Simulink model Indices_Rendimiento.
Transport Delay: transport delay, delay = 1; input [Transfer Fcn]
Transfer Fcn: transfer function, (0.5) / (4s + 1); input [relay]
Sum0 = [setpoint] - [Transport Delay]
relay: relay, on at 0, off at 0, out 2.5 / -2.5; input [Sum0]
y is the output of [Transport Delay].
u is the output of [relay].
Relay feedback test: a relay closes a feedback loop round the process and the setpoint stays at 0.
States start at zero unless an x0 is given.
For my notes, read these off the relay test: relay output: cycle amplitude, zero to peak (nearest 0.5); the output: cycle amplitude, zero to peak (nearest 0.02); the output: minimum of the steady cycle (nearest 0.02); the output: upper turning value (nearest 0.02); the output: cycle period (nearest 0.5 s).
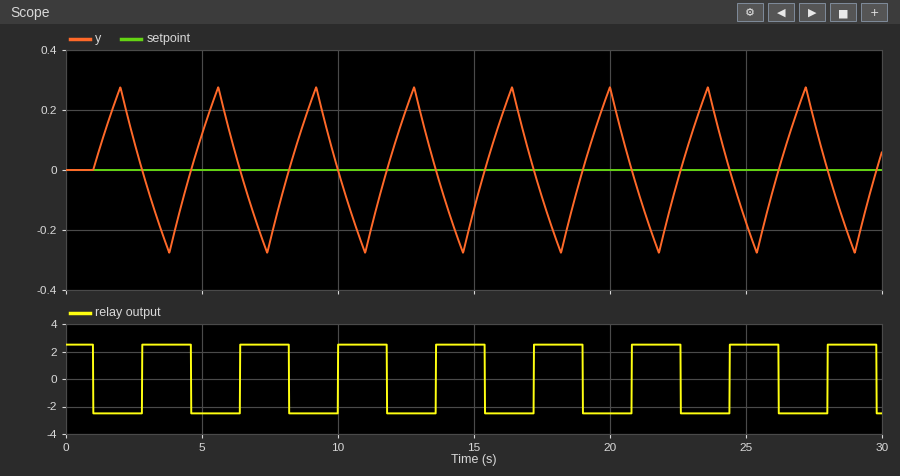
2.5
0.28
-0.28
0.28
3.5 s
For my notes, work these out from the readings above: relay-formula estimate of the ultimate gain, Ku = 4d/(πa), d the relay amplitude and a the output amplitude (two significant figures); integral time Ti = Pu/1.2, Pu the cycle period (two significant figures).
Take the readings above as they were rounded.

11
2.9 s
